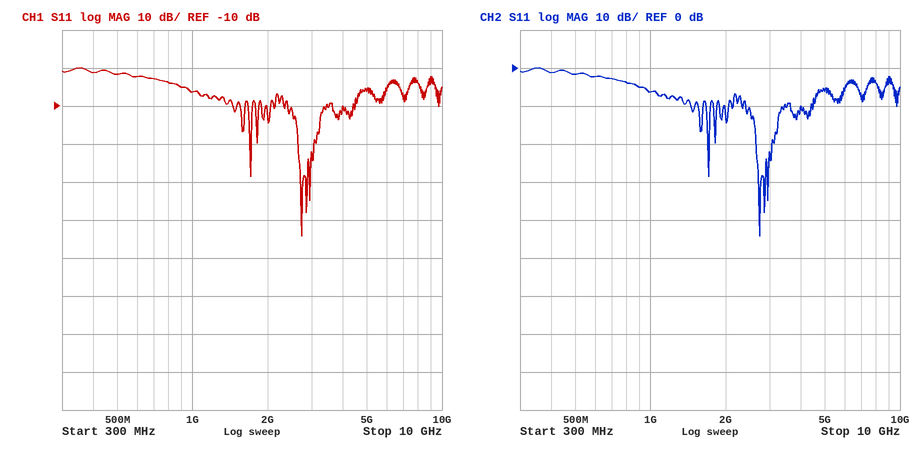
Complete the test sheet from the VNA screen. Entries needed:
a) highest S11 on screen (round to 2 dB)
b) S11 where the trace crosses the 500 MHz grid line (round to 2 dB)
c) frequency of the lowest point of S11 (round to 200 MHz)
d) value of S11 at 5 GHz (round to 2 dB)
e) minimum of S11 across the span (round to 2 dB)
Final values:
0 dB
-2 dB
2.8 GHz
-6 dB
-44 dB
